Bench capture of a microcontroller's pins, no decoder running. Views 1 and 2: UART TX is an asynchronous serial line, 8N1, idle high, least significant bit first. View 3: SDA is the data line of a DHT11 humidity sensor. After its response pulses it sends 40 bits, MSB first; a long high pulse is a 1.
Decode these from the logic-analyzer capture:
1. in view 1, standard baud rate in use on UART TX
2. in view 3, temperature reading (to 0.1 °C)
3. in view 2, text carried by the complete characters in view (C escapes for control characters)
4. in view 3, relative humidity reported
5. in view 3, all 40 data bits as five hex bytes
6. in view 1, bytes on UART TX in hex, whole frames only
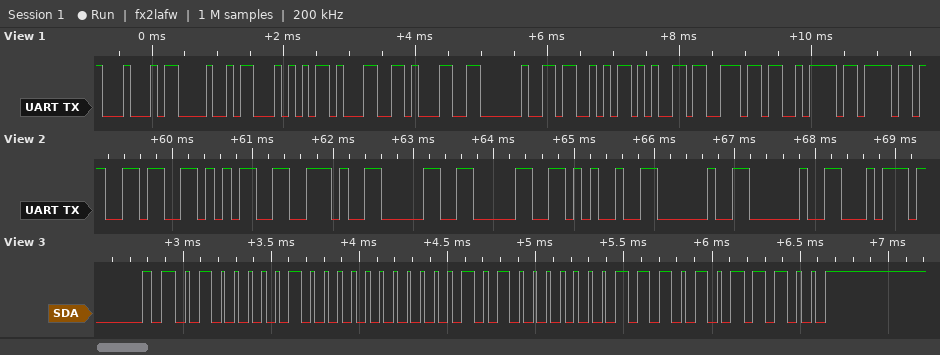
9600 baud
20.7 °C
"65.00%  t"
65 %
41 00 14 07 5C
44 48 54 31 31 20 53 65 6E 7A 6F
